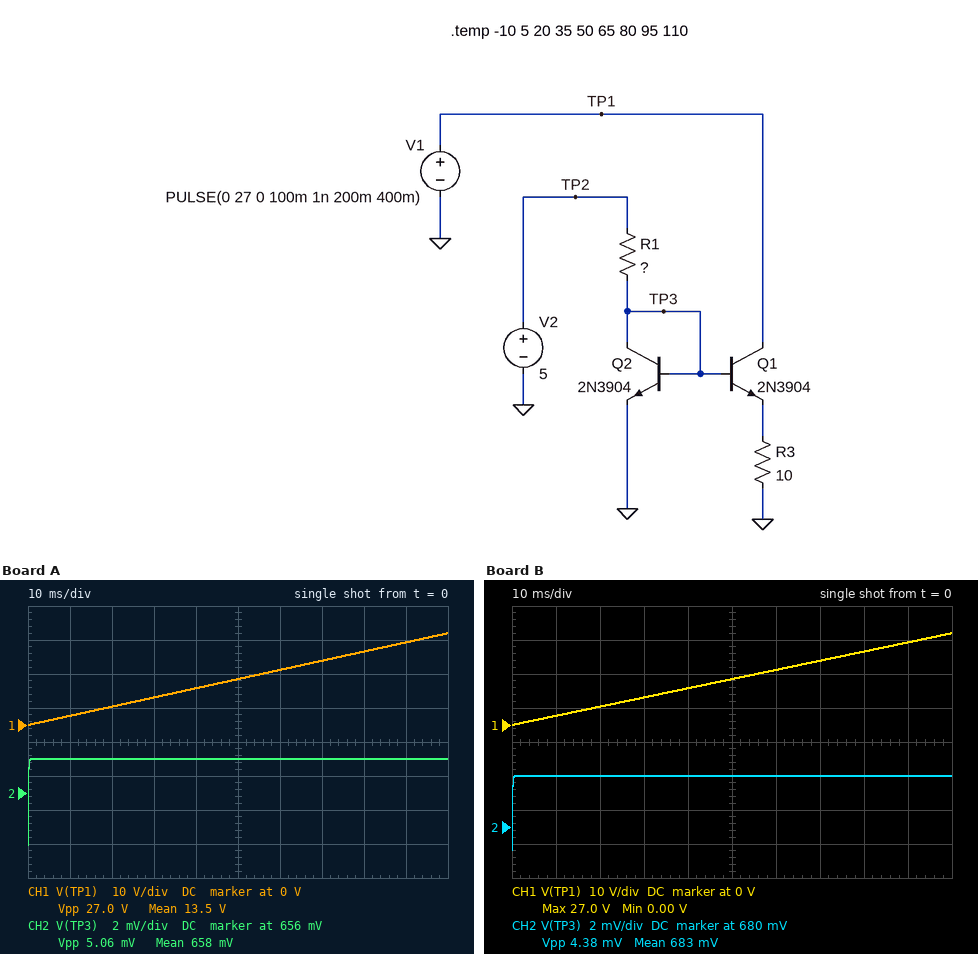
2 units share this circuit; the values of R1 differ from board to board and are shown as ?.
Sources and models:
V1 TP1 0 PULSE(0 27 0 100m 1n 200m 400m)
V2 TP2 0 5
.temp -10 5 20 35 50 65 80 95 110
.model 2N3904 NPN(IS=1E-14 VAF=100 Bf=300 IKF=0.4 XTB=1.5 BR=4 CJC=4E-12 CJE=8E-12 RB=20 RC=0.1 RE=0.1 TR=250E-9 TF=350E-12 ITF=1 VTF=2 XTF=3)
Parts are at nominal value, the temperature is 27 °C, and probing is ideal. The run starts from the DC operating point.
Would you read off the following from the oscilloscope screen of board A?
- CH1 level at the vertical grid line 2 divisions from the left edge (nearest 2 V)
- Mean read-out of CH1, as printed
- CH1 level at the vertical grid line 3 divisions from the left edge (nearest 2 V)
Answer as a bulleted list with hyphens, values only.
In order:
- 6 V
- 13.5 V
- 8 V
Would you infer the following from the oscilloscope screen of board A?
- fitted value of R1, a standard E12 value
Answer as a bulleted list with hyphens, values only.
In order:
- 3.9 kΩ
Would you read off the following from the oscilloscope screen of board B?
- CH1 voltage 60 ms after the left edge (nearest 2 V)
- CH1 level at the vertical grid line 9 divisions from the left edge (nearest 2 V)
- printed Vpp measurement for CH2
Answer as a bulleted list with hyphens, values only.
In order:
- 16 V
- 24 V
- 4.38 mV
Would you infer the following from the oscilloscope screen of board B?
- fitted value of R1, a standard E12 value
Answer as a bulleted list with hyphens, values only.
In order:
- 1.5 kΩ
